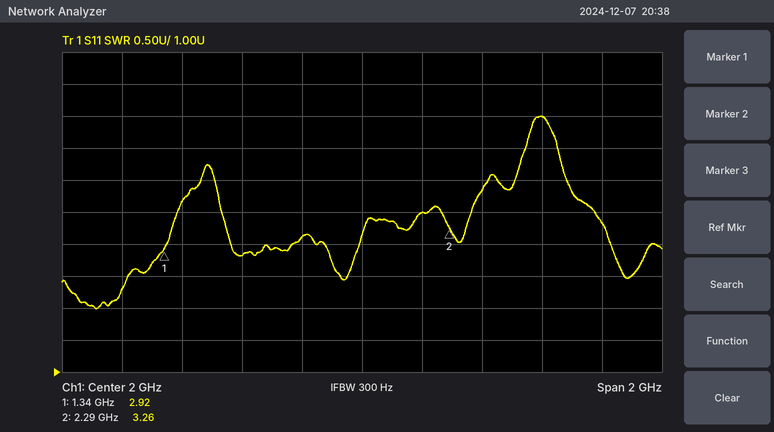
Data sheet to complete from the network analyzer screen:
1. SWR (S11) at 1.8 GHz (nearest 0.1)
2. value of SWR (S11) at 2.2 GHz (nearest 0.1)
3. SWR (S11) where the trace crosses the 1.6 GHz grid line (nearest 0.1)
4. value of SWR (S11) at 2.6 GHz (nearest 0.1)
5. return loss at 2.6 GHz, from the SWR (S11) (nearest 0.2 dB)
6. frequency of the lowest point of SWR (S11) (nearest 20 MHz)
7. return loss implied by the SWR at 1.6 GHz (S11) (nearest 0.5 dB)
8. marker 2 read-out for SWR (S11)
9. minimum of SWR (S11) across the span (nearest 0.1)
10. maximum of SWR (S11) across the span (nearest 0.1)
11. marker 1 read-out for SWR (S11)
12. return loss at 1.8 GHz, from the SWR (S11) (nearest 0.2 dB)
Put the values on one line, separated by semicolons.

3.1; 3.5; 2.8; 5.0; 3.6 dB; 1.12 GHz; 6.5 dB; 3.26; 2.0; 5.0; 2.92; 5.8 dB
